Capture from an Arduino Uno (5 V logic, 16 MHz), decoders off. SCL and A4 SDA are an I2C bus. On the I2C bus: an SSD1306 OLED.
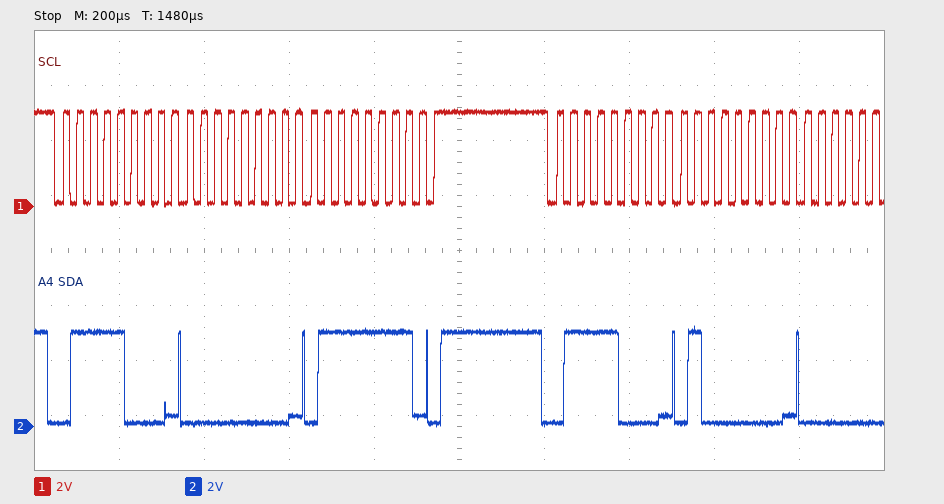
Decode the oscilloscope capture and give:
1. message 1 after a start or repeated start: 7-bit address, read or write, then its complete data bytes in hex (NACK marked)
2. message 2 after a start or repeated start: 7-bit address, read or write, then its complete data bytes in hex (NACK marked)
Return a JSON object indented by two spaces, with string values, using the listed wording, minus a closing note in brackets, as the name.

{
  "message 1 after a start or repeated start: 7-bit address, read or write, then its complete data bytes in hex": "0x3C write: 00 7F",
  "message 2 after a start or repeated start: 7-bit address, read or write, then its complete data bytes in hex": "0x3C write: 40"
}
